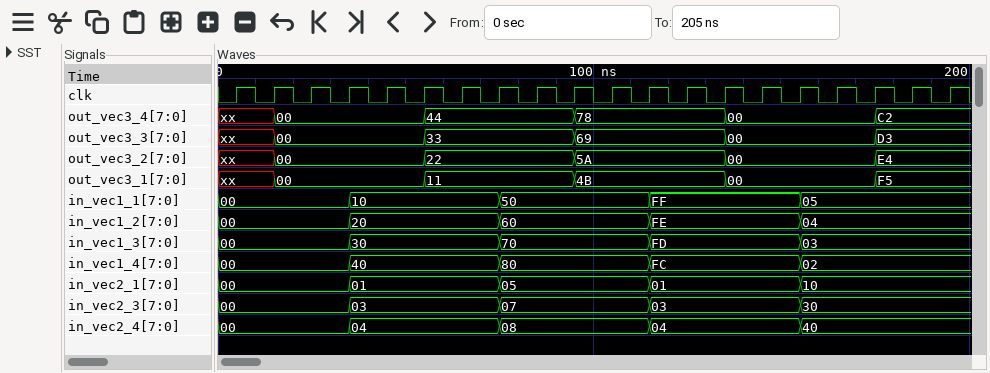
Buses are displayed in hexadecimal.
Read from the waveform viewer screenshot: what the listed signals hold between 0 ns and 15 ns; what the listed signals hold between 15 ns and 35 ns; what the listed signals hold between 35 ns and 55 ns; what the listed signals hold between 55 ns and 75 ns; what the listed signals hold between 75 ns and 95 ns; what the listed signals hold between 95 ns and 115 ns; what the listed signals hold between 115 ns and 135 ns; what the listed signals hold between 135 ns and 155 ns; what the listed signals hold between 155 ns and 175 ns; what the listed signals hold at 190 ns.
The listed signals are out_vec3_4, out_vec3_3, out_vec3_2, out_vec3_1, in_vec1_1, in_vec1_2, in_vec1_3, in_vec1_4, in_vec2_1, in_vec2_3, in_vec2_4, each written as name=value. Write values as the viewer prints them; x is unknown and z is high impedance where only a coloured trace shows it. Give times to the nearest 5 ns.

out_vec3_4=xx, out_vec3_3=xx, out_vec3_2=xx, out_vec3_1=xx, in_vec1_1=00, in_vec1_2=00, in_vec1_3=00, in_vec1_4=00, in_vec2_1=00, in_vec2_3=00, in_vec2_4=00
out_vec3_4=00, out_vec3_3=00, out_vec3_2=00, out_vec3_1=00, in_vec1_1=00, in_vec1_2=00, in_vec1_3=00, in_vec1_4=00, in_vec2_1=00, in_vec2_3=00, in_vec2_4=00
out_vec3_4=00, out_vec3_3=00, out_vec3_2=00, out_vec3_1=00, in_vec1_1=10, in_vec1_2=20, in_vec1_3=30, in_vec1_4=40, in_vec2_1=01, in_vec2_3=03, in_vec2_4=04
out_vec3_4=44, out_vec3_3=33, out_vec3_2=22, out_vec3_1=11, in_vec1_1=10, in_vec1_2=20, in_vec1_3=30, in_vec1_4=40, in_vec2_1=01, in_vec2_3=03, in_vec2_4=04
out_vec3_4=44, out_vec3_3=33, out_vec3_2=22, out_vec3_1=11, in_vec1_1=50, in_vec1_2=60, in_vec1_3=70, in_vec1_4=80, in_vec2_1=05, in_vec2_3=07, in_vec2_4=08
out_vec3_4=78, out_vec3_3=69, out_vec3_2=5A, out_vec3_1=4B, in_vec1_1=50, in_vec1_2=60, in_vec1_3=70, in_vec1_4=80, in_vec2_1=05, in_vec2_3=07, in_vec2_4=08
out_vec3_4=78, out_vec3_3=69, out_vec3_2=5A, out_vec3_1=4B, in_vec1_1=FF, in_vec1_2=FE, in_vec1_3=FD, in_vec1_4=FC, in_vec2_1=01, in_vec2_3=03, in_vec2_4=04
out_vec3_4=00, out_vec3_3=00, out_vec3_2=00, out_vec3_1=00, in_vec1_1=FF, in_vec1_2=FE, in_vec1_3=FD, in_vec1_4=FC, in_vec2_1=01, in_vec2_3=03, in_vec2_4=04
out_vec3_4=00, out_vec3_3=00, out_vec3_2=00, out_vec3_1=00, in_vec1_1=05, in_vec1_2=04, in_vec1_3=03, in_vec1_4=02, in_vec2_1=10, in_vec2_3=30, in_vec2_4=40
out_vec3_4=C2, out_vec3_3=D3, out_vec3_2=E4, out_vec3_1=F5, in_vec1_1=05, in_vec1_2=04, in_vec1_3=03, in_vec1_4=02, in_vec2_1=10, in_vec2_3=30, in_vec2_4=40
